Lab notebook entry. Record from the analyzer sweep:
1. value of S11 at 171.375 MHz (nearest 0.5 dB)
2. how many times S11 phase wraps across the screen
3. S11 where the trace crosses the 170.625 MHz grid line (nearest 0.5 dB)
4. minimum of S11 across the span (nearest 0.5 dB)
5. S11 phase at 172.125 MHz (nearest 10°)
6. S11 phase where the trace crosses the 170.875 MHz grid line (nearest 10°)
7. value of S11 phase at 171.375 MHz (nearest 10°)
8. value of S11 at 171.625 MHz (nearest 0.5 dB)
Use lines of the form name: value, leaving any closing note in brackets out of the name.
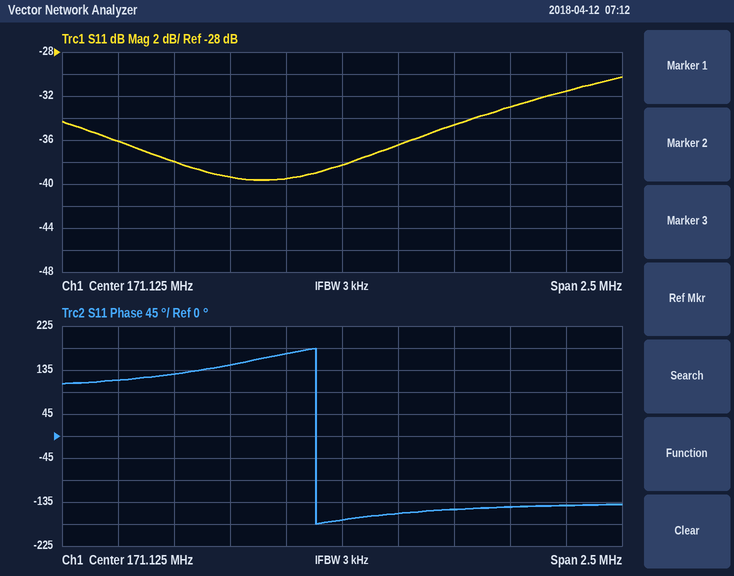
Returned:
value of S11 at 171.375 MHz: -36.5 dB
how many times S11 phase wraps across the screen: 1
S11 where the trace crosses the 170.625 MHz grid line: -39.5 dB
minimum of S11 across the span: -39.5 dB
S11 phase at 172.125 MHz: -140°
S11 phase where the trace crosses the 170.875 MHz grid line: 170°
value of S11 phase at 171.375 MHz: -160°
value of S11 at 171.625 MHz: -34.5 dB
